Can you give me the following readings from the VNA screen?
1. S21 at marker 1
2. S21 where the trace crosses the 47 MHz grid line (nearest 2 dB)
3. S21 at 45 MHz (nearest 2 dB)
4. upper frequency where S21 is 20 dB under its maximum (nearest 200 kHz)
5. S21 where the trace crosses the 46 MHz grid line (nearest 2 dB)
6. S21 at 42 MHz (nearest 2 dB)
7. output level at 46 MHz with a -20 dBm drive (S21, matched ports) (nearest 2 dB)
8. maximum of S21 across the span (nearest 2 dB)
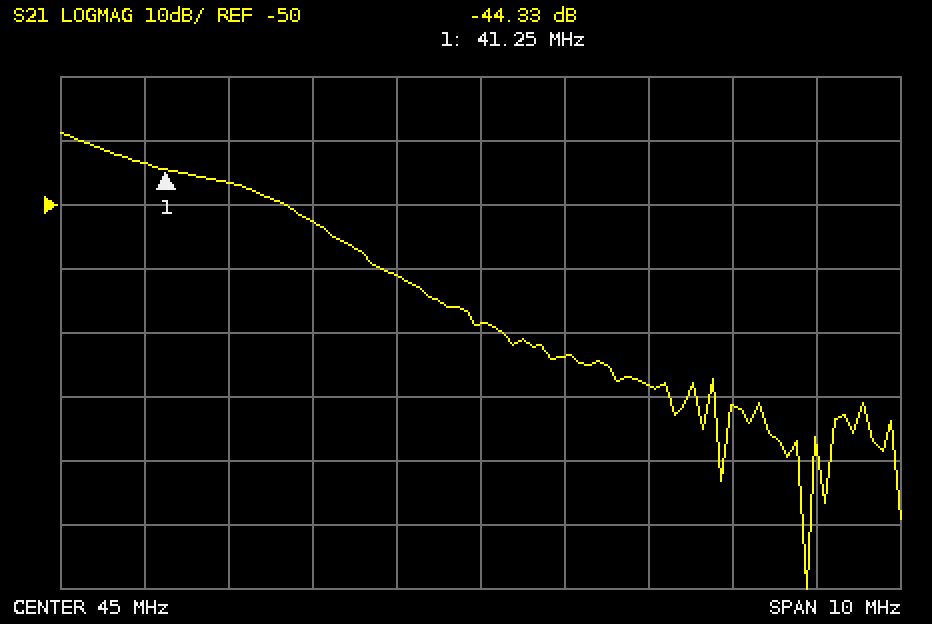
-44.33 dB
-78 dB
-68 dB
43.6 MHz
-74 dB
-46 dB
-94 dBm
-38 dB
